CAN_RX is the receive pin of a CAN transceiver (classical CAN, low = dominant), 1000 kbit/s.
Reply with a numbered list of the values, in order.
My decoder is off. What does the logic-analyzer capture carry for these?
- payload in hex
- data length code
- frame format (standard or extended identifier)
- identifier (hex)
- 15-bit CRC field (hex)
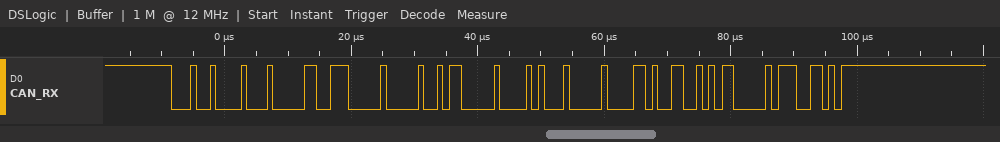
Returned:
1. 27 00 0B 00 51 00 69 95
2. 8
3. standard
4. 0x121
5. 0x40E6
